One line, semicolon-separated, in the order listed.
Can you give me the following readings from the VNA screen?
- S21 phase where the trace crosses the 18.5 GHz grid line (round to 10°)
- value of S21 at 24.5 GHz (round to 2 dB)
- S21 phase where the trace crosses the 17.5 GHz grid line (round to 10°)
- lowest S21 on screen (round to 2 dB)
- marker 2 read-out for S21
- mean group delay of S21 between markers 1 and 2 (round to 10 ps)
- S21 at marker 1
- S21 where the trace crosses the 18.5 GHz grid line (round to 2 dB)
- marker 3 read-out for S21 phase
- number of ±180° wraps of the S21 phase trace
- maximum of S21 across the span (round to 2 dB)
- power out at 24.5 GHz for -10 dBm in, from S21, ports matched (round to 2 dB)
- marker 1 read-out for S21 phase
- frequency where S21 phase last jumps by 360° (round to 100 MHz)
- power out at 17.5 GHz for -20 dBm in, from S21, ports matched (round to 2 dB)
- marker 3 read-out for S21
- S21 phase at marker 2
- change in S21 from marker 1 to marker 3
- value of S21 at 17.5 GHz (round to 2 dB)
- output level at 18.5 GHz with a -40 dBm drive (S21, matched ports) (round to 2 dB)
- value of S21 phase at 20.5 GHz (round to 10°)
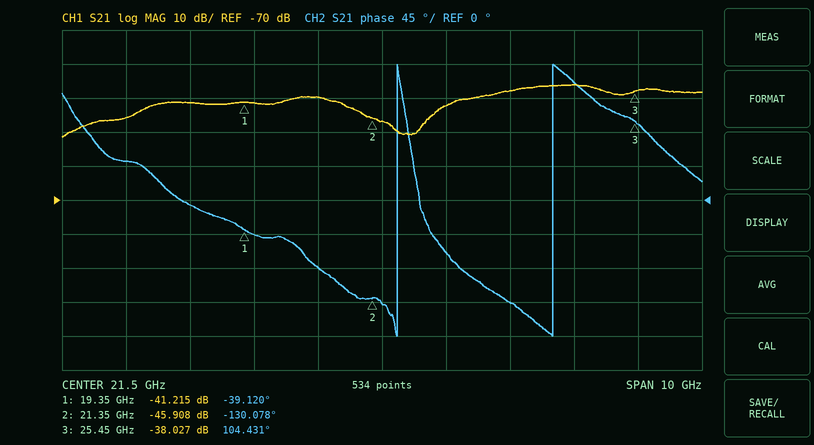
-10°; -36 dB; 50°; -52 dB; -45.908 dB; 130 ps; -41.215 dB; -42 dB; 104.431°; 2; -36 dB; -46 dBm; -39.120°; 24.2 GHz; -66 dBm; -38.027 dB; -130.078°; 3.188 dB; -46 dB; -82 dBm; -90°
